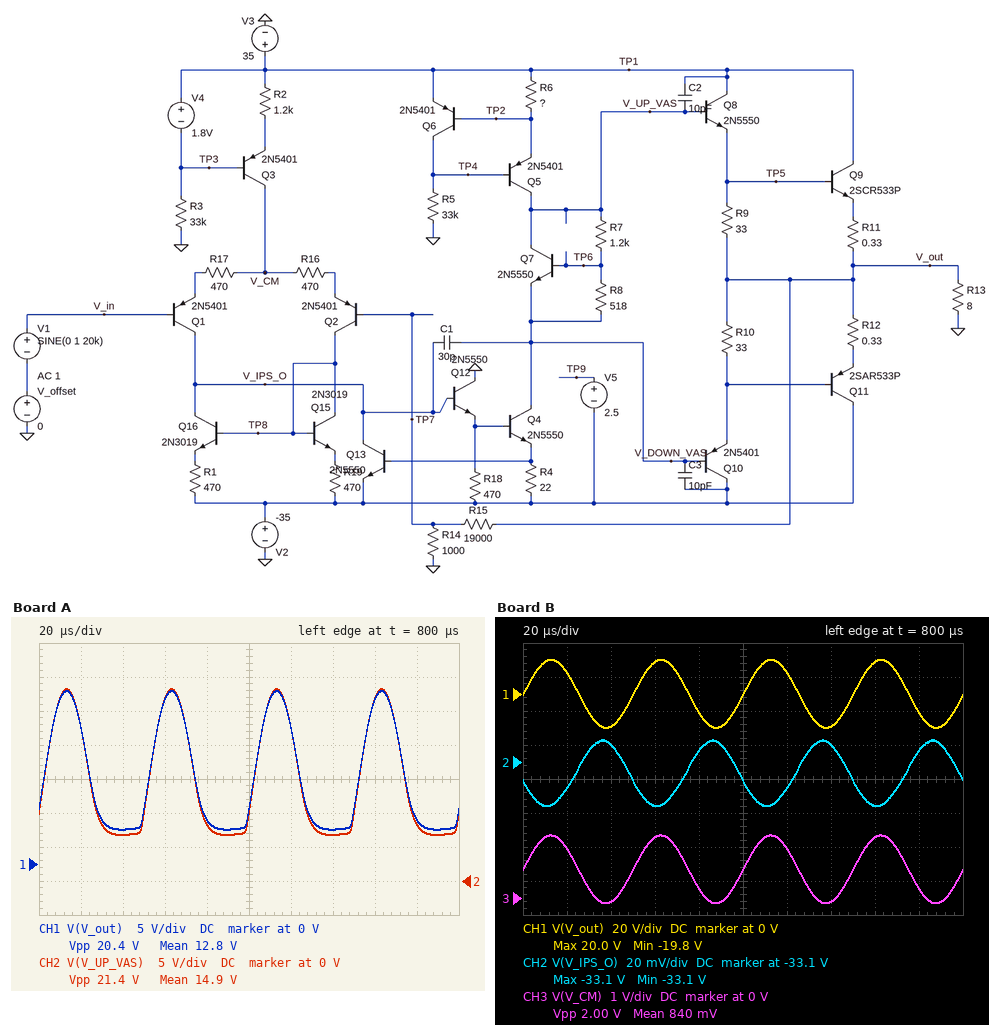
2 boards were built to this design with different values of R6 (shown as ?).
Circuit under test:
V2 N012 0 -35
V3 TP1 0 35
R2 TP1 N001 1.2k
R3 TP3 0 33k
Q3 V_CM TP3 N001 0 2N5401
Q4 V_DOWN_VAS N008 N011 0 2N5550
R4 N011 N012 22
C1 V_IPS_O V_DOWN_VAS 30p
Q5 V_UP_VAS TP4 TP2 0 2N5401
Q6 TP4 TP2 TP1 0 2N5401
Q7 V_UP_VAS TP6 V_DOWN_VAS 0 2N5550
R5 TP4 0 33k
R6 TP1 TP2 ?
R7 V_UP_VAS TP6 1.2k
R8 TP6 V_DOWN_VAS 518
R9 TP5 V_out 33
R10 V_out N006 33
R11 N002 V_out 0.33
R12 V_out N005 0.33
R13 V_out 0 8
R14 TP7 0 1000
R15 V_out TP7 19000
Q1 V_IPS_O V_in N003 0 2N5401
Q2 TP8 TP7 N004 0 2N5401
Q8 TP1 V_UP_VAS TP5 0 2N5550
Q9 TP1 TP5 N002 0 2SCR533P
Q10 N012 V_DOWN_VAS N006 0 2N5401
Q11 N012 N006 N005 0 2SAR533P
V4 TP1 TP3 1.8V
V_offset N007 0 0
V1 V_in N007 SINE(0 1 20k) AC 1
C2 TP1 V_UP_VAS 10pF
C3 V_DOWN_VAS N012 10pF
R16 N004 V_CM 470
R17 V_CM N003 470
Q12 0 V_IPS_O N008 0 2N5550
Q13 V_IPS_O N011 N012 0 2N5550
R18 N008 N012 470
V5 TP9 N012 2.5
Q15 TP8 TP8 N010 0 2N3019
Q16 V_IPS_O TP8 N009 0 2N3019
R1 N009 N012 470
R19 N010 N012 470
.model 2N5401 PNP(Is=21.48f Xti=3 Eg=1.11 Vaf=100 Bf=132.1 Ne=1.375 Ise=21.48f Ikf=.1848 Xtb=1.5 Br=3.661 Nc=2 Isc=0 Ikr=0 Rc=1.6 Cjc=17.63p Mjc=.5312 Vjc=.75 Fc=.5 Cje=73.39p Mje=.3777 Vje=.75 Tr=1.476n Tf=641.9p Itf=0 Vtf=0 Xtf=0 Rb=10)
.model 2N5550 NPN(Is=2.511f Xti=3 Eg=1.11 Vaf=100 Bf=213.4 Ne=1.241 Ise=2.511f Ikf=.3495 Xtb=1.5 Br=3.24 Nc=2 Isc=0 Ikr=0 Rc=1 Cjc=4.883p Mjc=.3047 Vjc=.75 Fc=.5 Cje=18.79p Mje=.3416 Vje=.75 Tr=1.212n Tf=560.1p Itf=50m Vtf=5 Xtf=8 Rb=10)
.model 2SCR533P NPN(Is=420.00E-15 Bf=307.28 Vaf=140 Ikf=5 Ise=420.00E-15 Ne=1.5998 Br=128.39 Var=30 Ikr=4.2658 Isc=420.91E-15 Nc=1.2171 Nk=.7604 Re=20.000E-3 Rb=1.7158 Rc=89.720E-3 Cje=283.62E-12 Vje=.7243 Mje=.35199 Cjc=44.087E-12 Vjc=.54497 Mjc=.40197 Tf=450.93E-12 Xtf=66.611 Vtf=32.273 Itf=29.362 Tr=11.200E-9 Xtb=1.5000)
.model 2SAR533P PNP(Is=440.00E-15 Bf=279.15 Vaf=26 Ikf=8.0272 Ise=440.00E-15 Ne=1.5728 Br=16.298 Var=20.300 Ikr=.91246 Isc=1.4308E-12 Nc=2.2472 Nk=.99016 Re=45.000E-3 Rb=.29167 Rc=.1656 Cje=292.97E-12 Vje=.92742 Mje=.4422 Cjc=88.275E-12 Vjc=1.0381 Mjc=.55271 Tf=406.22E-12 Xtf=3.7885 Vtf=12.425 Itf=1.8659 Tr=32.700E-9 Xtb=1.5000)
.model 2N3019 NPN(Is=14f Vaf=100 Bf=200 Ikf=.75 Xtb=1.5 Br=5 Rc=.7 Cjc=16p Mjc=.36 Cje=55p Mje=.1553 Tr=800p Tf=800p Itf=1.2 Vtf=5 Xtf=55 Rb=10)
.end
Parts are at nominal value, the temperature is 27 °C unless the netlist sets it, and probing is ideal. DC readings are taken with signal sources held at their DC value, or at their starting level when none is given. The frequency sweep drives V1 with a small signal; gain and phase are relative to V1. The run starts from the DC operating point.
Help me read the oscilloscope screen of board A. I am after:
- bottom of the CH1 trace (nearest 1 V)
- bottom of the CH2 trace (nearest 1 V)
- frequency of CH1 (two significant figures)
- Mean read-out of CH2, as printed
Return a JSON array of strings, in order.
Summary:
["5 V", "7 V", "20 kHz", "14.9 V"]
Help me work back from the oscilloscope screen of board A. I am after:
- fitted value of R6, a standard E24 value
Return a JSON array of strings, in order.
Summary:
["20 Ω"]
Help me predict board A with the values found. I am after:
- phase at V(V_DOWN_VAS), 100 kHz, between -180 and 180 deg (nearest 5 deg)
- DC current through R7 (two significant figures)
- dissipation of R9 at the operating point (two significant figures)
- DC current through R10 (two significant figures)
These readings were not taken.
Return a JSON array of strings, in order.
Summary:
["-30 deg", "1.7 mA", "41 mW", "7.5 mA"]
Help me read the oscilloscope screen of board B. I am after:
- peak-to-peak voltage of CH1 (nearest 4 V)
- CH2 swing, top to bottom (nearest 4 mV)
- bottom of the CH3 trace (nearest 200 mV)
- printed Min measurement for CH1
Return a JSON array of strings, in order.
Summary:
["40 V", "40 mV", "-200 mV", "-19.8 V"]
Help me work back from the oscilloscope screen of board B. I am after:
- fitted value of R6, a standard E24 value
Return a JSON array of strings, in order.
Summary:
["33 Ω"]
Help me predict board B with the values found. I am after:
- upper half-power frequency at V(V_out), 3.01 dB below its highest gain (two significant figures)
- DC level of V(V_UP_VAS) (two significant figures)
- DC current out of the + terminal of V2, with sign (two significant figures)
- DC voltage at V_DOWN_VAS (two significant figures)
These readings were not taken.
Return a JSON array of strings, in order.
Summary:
["490 kHz", "1.5 V", "-52 mA", "-1.2 V"]
